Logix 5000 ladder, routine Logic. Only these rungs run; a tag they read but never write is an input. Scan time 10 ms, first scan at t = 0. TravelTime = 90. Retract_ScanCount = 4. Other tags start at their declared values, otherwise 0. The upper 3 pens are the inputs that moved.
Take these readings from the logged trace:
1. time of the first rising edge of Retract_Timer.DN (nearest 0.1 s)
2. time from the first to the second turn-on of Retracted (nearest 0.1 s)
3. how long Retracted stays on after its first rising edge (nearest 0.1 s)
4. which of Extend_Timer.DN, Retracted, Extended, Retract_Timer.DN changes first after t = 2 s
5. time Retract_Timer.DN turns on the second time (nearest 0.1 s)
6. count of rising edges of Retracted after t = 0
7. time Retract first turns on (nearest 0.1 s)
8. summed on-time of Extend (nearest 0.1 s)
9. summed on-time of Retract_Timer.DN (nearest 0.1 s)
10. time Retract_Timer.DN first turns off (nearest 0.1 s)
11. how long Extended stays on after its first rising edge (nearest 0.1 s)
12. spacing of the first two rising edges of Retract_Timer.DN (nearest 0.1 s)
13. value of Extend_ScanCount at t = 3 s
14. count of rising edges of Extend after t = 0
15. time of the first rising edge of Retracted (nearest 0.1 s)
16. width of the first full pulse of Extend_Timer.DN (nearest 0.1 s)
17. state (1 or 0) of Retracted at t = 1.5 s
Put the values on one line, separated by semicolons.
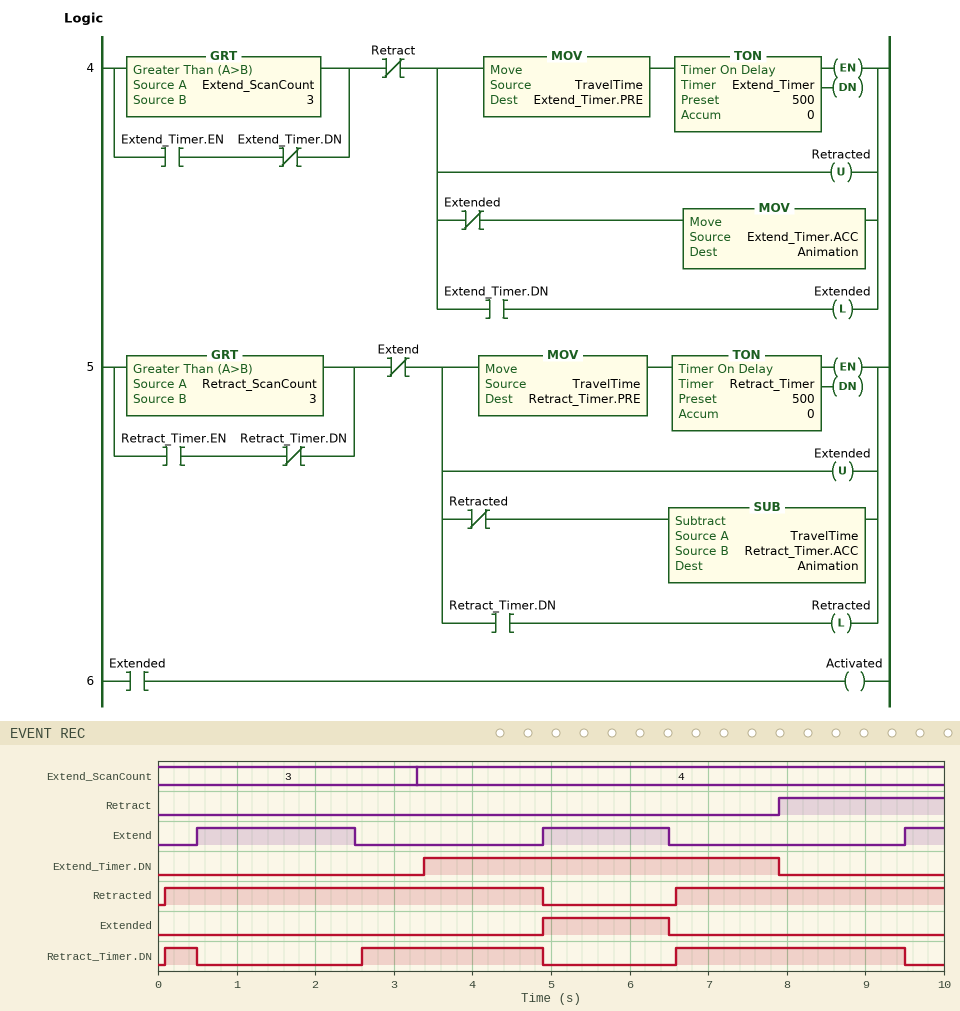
0.1 s; 6.5 s; 4.8 s; Retract_Timer.DN; 2.6 s; 2; 7.9 s; 4.1 s; 5.6 s; 0.5 s; 1.6 s; 2.5 s; 3; 3; 0.1 s; 4.5 s; 1
